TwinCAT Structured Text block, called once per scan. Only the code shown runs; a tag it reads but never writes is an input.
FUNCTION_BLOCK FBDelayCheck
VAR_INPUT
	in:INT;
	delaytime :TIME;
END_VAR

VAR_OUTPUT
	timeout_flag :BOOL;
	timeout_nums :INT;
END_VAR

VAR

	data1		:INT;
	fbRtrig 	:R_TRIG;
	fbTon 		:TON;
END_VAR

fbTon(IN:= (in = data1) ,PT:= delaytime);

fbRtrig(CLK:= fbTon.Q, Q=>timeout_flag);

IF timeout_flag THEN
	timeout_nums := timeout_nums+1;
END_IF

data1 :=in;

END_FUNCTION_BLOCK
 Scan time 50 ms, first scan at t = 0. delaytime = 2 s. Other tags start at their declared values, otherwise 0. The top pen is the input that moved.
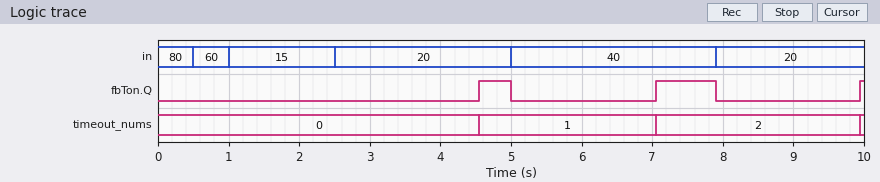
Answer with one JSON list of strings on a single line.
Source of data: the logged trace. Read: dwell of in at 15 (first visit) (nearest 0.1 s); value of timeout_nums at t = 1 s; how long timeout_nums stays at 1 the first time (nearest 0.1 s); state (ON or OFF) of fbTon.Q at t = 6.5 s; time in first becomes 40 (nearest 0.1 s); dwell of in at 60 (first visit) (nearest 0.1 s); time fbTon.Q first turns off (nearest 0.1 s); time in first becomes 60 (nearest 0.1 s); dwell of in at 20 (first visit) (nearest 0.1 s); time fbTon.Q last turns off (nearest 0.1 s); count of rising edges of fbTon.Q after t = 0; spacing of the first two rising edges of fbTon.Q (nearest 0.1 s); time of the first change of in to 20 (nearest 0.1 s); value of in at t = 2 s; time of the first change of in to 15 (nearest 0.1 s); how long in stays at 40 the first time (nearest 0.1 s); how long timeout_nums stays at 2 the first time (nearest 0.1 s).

["1.5 s", "0", "2.5 s", "OFF", "5.0 s", "0.5 s", "5.0 s", "0.5 s", "2.5 s", "7.9 s", "3", "2.5 s", "2.5 s", "15", "1.0 s", "2.9 s", "2.9 s"]
